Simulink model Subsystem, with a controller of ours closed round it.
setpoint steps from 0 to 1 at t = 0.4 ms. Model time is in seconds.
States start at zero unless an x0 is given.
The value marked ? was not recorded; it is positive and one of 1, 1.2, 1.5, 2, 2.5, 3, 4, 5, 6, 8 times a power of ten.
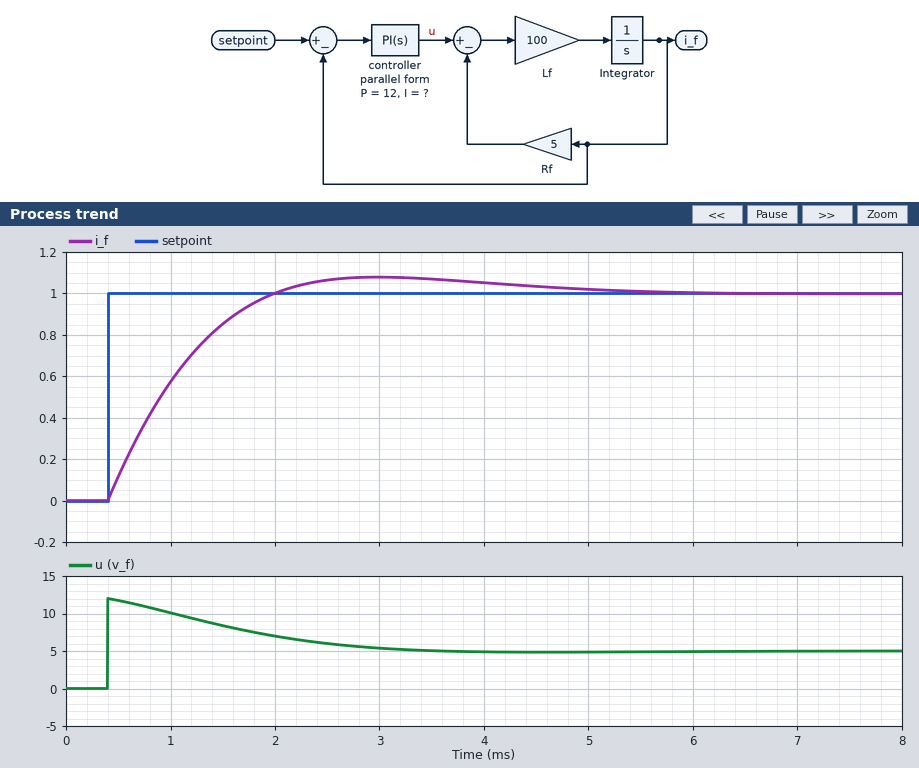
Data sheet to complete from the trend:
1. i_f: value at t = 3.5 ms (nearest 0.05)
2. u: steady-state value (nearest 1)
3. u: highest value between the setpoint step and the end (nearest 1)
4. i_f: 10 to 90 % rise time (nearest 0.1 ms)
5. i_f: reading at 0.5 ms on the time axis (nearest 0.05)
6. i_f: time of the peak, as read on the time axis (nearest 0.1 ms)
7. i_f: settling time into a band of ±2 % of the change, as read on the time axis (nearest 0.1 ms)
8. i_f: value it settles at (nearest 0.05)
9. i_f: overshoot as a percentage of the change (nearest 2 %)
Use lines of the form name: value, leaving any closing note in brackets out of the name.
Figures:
i_f: value at t = 3.5 ms: 1.05
u: steady-state value: 5
u: highest value between the setpoint step and the end: 12
i_f: 10 to 90 % rise time: 1.1 ms
i_f: reading at 0.5 ms on the time axis: 0.10
i_f: time of the peak, as read on the time axis: 3.0 ms
i_f: settling time into a band of ±2 % of the change, as read on the time axis: 5.0 ms
i_f: value it settles at: 1.00
i_f: overshoot as a percentage of the change: 8 %
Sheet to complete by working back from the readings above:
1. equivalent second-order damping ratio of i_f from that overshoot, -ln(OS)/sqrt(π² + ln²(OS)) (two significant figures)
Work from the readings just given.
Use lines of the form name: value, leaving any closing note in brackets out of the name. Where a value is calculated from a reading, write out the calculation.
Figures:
equivalent second-order damping ratio of i_f from that overshoot, -ln(OS)/sqrt(π² + ln²(OS)): ln(0.08) = -2.526; 2.526 / sqrt(9.870 + 6.379) = 0.63
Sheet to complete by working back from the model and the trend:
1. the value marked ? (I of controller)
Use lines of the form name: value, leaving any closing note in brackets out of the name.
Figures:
the value marked ?: 12000
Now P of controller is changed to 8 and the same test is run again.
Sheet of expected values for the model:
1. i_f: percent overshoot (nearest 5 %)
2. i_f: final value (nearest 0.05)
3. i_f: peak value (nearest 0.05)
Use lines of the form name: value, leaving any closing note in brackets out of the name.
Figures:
i_f: percent overshoot: 15 %
i_f: final value: 1.00
i_f: peak value: 1.15
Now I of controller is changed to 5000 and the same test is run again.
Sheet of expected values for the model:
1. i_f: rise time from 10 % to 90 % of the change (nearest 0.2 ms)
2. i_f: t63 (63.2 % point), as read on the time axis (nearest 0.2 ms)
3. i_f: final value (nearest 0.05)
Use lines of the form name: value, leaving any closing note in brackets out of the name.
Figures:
i_f: rise time from 10 % to 90 % of the change: 2.2 ms
i_f: t63 (63.2 % point), as read on the time axis: 1.2 ms
i_f: final value: 1.00
